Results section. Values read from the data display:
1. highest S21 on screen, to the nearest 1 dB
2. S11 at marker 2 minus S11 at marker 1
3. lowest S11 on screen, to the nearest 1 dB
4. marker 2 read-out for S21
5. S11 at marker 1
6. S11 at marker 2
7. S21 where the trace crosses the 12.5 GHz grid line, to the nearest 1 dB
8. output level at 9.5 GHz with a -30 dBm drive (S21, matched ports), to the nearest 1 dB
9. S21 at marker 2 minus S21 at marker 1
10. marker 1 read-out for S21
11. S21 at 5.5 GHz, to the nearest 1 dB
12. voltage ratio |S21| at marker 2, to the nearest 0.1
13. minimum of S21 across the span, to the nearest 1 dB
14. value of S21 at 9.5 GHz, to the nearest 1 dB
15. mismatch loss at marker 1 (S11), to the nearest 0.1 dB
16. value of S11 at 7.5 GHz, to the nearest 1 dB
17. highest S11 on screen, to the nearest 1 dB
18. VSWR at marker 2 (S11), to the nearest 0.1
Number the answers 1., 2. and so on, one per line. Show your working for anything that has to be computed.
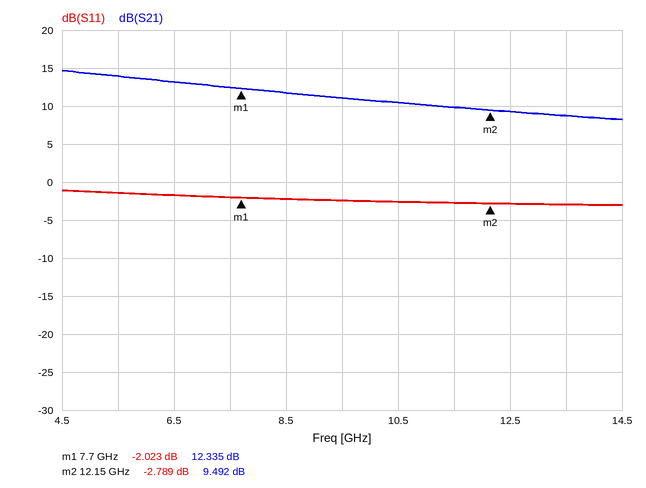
1. 15 dB
2. -2.789 − (-2.023) = -0.766 dB
3. -3 dB
4. 9.492 dB
5. -2.023 dB
6. -2.789 dB
7. 9 dB
8. -30 dBm + (11 dB) = -19 dBm
9. 9.492 − (12.335) = -2.843 dB
10. 12.335 dB
11. 14 dB
12. 10^(9.492/20) ≈ 3.0
13. 8 dB
14. 11 dB
15. −10 log10(1 − 10^(-2.023/10)) ≈ 4.3 dB
16. -2 dB
17. -1 dB
18. (1 + 0.7254)/(1 − 0.7254) ≈ 6.3
